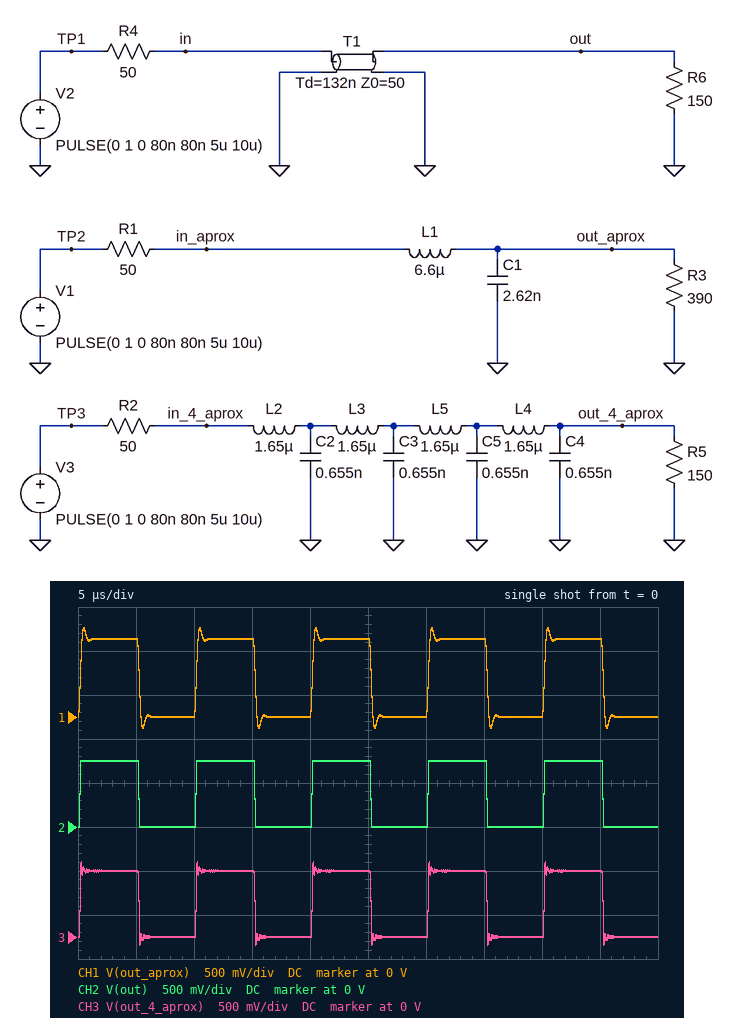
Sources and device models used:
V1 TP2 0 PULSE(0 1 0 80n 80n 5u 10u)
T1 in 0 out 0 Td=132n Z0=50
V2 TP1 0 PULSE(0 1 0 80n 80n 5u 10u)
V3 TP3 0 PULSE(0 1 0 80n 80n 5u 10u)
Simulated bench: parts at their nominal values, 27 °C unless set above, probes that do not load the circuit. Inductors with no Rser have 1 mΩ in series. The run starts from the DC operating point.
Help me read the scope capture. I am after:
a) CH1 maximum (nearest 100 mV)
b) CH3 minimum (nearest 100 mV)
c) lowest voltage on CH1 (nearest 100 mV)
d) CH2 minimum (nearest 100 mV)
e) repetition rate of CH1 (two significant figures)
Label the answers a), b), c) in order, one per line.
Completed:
a) 1.0 V
b) -100 mV
c) -100 mV
d) 0 V
e) 100 kHz
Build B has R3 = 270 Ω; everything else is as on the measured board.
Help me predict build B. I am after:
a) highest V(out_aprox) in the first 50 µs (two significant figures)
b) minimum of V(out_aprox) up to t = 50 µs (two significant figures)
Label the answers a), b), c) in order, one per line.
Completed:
a) 950 mV
b) -110 mV
